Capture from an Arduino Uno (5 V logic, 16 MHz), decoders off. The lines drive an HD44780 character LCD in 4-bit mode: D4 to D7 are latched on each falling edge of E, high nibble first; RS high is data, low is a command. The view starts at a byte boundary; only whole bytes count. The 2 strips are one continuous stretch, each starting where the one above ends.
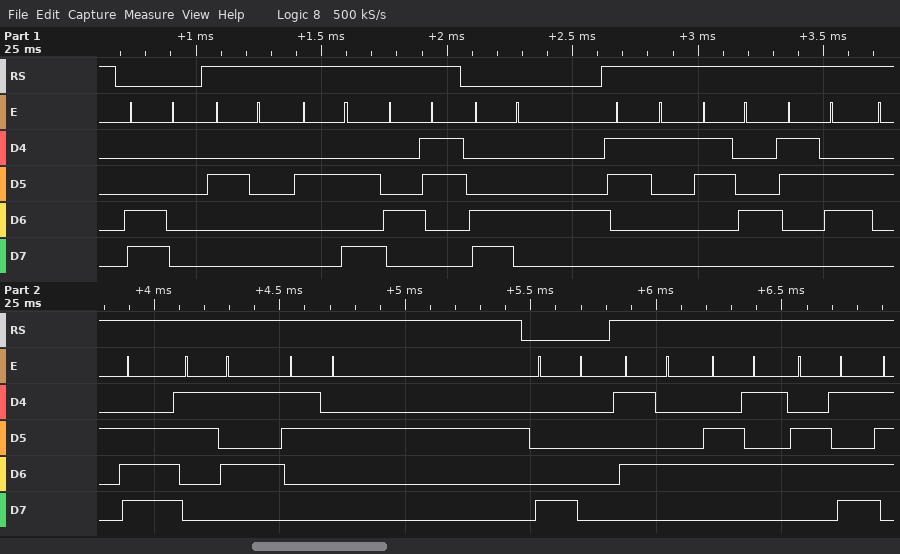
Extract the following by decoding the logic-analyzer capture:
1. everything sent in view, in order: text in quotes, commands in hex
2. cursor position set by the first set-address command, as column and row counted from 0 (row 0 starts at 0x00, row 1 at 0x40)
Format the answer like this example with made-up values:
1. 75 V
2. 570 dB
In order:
1. 0xC0 " *C" 0xC4 "146.52" 0x80 "Tem"
2. column 0, row 1
